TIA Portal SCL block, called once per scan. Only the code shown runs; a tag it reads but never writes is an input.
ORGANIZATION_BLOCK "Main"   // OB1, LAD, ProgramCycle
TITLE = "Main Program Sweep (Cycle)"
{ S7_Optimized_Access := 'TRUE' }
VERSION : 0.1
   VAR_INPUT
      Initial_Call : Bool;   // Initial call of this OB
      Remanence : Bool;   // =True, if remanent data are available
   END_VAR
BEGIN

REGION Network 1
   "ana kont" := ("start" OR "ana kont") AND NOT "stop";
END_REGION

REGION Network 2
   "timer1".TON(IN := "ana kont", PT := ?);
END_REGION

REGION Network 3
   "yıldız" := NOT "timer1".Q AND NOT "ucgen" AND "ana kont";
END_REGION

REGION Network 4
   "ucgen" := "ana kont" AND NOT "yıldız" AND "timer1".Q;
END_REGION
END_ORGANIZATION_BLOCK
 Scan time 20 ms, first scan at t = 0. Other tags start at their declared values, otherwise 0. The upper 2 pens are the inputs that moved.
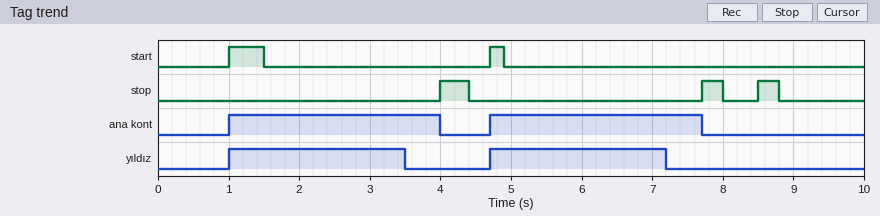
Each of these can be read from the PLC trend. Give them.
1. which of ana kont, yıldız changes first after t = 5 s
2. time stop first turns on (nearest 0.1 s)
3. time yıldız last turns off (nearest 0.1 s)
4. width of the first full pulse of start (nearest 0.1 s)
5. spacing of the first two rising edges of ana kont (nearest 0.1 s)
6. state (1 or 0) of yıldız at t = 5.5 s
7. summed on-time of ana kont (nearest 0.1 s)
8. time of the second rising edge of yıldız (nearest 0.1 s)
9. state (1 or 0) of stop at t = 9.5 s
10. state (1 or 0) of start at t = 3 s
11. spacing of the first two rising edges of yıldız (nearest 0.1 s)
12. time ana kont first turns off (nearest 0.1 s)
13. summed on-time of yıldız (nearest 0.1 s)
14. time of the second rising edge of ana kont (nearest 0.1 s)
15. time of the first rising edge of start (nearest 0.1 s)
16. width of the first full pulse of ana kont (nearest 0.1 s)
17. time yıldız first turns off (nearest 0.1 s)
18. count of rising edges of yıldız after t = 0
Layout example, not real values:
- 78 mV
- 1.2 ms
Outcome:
- yıldız
- 4.0 s
- 7.2 s
- 0.5 s
- 3.7 s
- 1
- 6.0 s
- 4.7 s
- 0
- 0
- 3.7 s
- 4.0 s
- 5.0 s
- 4.7 s
- 1.0 s
- 3.0 s
- 3.5 s
- 2
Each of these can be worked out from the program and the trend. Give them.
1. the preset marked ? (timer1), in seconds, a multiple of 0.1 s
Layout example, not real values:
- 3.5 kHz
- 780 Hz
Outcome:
- 2.5 s
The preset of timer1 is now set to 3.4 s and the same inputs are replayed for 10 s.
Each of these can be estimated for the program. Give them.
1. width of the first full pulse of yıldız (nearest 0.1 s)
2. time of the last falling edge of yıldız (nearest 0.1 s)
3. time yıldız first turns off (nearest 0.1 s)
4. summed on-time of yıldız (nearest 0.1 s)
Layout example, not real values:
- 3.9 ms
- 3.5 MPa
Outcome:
- 3.0 s
- 7.7 s
- 4.0 s
- 6.0 s
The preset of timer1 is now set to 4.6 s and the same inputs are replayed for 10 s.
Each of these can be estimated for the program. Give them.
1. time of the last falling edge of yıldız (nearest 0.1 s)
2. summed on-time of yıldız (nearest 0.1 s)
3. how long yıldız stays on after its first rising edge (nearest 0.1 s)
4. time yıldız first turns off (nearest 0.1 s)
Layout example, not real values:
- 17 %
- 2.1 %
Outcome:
- 7.7 s
- 6.0 s
- 3.0 s
- 4.0 s
